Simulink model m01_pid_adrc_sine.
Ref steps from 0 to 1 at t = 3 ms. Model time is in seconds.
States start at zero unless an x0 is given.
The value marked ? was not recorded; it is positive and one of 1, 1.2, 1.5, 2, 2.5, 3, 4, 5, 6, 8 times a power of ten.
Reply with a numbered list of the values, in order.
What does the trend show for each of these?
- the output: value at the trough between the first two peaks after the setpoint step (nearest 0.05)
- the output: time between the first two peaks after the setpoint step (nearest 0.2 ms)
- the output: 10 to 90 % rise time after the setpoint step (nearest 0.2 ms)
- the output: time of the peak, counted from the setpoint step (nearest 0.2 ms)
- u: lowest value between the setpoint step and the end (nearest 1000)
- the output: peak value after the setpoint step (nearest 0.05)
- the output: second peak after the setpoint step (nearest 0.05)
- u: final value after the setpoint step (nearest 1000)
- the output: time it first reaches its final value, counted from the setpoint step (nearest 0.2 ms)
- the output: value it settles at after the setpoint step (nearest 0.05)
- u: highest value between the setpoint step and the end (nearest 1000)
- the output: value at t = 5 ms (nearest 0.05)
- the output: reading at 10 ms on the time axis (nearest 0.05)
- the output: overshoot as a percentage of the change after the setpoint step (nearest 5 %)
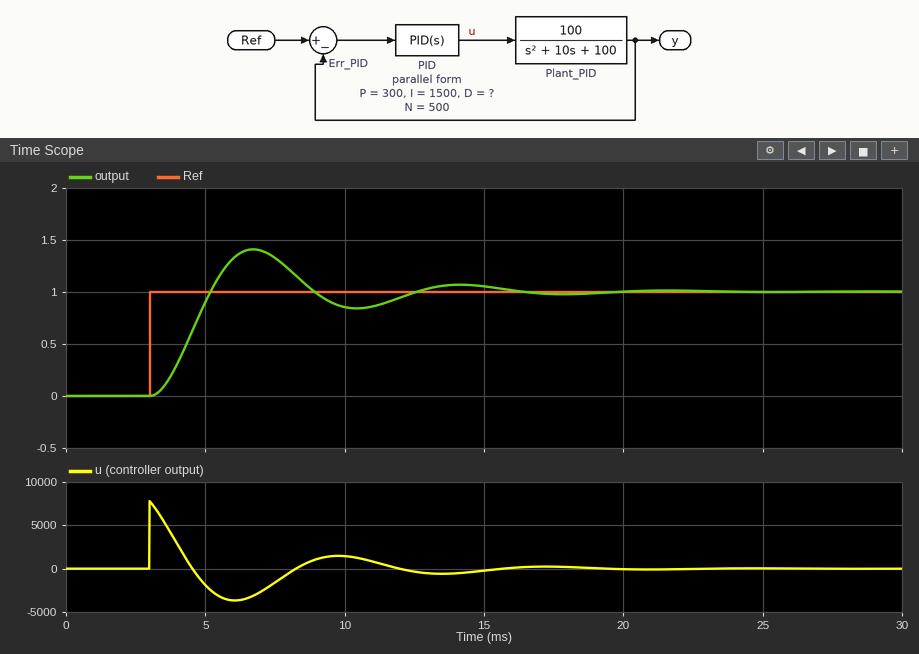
1. 0.85
2. 7.4 ms
3. 1.4 ms
4. 3.8 ms
5. -4000
6. 1.40
7. 1.05
8. 0
9. 2.2 ms
10. 1.00
11. 8000
12. 0.90
13. 0.85
14. 40 %
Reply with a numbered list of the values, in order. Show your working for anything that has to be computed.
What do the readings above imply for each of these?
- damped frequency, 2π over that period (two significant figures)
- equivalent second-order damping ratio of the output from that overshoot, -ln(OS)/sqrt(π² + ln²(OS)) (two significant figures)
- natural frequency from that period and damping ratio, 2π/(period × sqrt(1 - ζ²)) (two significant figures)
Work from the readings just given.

1. 2π / 7.4 = 0.85 rad/ms
2. ln(0.4) = -0.916; 0.916 / sqrt(9.870 + 0.840) = 0.28
3. 2π / (7.4 × sqrt(1 - 0.28²)) = 0.88 rad/ms
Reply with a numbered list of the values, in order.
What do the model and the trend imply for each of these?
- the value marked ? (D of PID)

1. 15
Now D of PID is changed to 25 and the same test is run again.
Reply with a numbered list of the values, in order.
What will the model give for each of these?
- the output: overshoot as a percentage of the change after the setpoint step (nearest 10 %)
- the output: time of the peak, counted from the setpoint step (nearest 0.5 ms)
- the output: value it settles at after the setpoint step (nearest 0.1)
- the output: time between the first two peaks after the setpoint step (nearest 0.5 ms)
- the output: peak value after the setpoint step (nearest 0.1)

1. 50 %
2. 3.0 ms
3. 1.0
4. 5.5 ms
5. 1.5
